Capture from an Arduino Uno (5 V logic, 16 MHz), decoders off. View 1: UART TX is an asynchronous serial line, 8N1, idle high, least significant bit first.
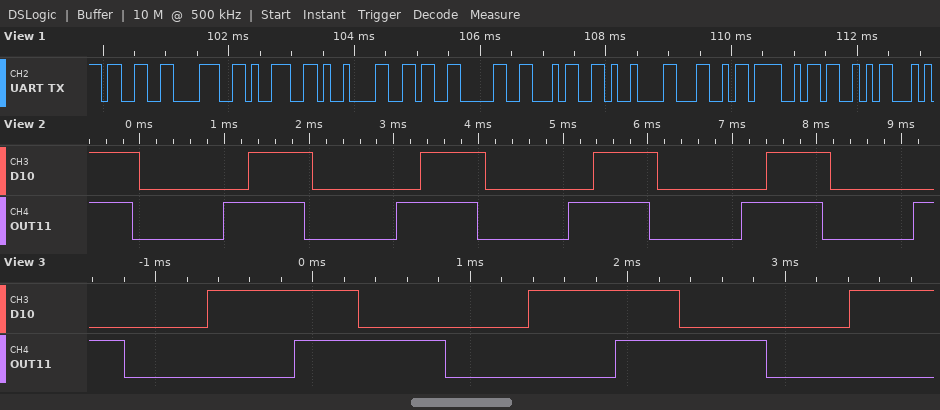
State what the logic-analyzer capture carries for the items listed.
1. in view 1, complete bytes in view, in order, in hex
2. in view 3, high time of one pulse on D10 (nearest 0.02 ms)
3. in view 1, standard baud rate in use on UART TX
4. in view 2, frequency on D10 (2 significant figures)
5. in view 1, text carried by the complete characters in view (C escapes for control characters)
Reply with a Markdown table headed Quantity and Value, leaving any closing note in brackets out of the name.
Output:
| Quantity | Value |
|---|---|
| in view 1, complete bytes in view, in order, in hex | 33 38 39 09 36 30 34 09 4C 4F 53 |
| in view 3, high time of one pulse on D10 | 0.96 ms |
| in view 1, standard baud rate in use on UART TX | 9600 baud |
| in view 2, frequency on D10 | 490 Hz |
| in view 1, text carried by the complete characters in view | "389\t604\tLOS" |
